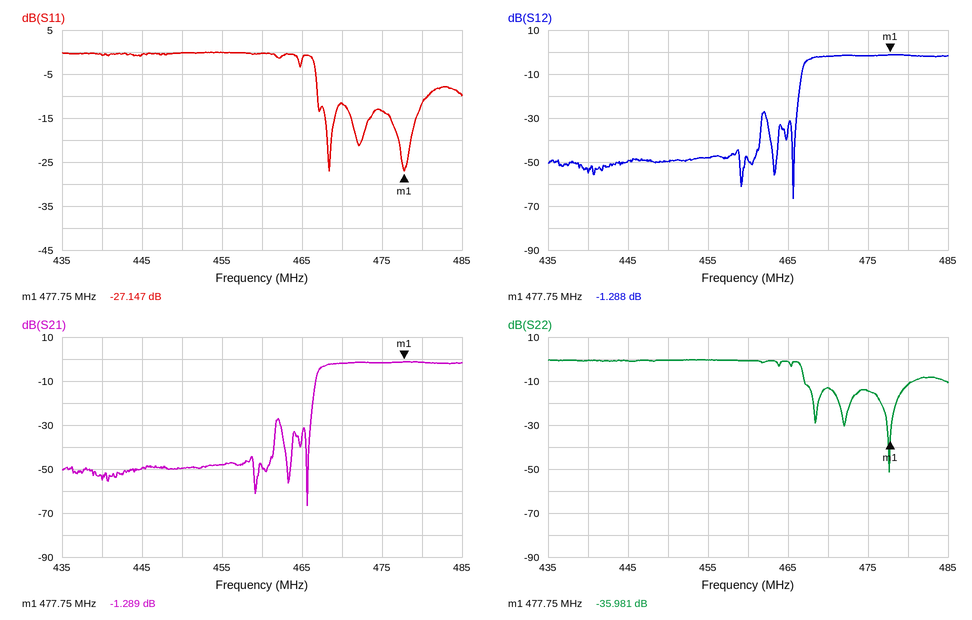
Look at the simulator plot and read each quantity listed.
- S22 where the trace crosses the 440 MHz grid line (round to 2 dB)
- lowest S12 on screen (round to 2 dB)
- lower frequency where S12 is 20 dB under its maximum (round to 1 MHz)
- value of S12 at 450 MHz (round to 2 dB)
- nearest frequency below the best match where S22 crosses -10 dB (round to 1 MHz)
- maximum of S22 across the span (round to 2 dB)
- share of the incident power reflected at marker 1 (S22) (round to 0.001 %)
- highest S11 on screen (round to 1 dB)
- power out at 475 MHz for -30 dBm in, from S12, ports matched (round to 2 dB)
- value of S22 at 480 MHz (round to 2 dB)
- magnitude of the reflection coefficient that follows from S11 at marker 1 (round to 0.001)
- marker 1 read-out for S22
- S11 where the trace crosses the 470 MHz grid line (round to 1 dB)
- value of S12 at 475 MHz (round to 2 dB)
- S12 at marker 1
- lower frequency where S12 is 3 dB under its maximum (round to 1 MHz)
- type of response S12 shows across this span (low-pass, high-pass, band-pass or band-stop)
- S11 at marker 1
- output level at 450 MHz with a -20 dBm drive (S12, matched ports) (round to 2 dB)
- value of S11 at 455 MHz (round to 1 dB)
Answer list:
0 dB
-66 dB
466 MHz
-50 dB
467 MHz
0 dB
0.025 %
0 dB
-32 dBm
-12 dB
0.044
-35.981 dB
-12 dB
-2 dB
-1.288 dB
467 MHz
high-pass
-27.147 dB
-70 dBm
0 dB
